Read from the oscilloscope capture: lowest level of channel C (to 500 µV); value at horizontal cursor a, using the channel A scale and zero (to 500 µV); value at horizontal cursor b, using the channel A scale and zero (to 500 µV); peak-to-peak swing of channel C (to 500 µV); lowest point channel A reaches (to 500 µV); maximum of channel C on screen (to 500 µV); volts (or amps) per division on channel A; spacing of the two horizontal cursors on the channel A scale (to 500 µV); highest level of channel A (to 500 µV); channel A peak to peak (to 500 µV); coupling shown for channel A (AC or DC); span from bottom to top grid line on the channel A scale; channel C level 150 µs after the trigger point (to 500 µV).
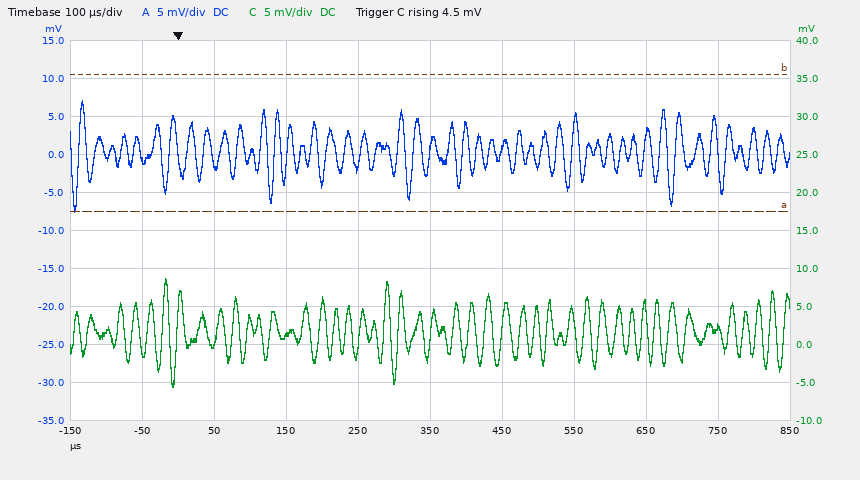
-5.5 mV
-7.5 mV
10.5 mV
14.0 mV
-7.5 mV
8.5 mV
5 mV
18.0 mV
7.0 mV
14.5 mV
DC
50 mV
1.0 mV
